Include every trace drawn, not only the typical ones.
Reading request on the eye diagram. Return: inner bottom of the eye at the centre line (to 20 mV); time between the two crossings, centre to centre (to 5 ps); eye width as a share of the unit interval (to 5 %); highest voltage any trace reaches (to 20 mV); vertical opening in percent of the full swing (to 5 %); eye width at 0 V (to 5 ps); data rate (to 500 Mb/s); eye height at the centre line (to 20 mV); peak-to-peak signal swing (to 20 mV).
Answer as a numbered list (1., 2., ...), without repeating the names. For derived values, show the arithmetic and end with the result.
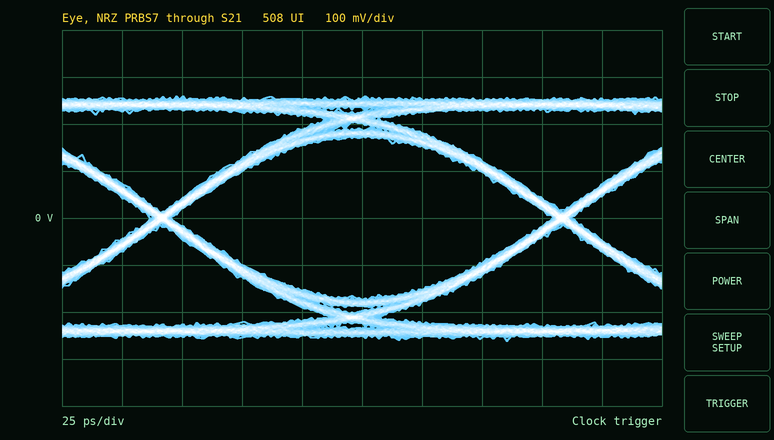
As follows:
1. -180 mV
2. 165 ps
3. 160 ps / 165 ps ≈ 97.0 %, so 95 % to the nearest 5 %
4. 260 mV
5. 340 mV / 520 mV ≈ 65 %
6. 160 ps
7. 6.0 Gb/s
8. 340 mV
9. 520 mV
